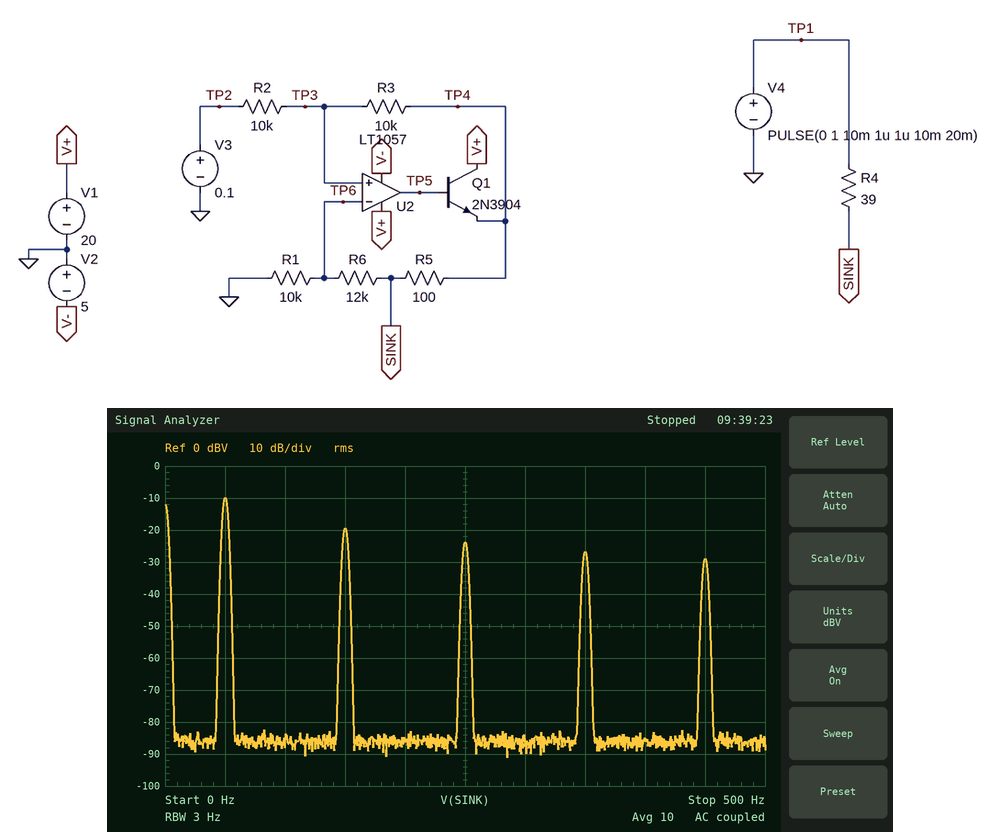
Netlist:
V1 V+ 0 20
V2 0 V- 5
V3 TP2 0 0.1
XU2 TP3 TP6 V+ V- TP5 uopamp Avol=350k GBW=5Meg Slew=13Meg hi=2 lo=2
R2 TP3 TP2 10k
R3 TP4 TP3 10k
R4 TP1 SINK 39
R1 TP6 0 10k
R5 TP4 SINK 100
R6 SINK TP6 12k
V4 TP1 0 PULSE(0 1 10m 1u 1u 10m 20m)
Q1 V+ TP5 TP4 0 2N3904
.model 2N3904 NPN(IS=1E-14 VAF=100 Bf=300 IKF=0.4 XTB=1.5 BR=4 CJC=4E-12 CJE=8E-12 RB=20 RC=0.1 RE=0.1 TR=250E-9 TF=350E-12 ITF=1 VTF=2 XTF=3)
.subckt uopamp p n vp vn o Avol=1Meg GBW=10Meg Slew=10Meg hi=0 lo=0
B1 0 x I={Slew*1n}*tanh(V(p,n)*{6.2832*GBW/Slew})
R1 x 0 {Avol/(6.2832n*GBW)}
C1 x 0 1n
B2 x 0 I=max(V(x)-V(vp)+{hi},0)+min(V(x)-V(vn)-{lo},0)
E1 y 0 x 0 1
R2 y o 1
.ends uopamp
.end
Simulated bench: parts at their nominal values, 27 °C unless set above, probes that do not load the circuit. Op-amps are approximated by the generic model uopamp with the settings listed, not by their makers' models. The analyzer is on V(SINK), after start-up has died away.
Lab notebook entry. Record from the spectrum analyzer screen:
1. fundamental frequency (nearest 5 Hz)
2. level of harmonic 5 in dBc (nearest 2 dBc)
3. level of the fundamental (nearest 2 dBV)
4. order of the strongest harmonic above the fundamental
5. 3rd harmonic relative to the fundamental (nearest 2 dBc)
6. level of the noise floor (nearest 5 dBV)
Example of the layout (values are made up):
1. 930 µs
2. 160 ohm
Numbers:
1. 50 Hz
2. -14 dBc
3. -10 dBV
4. 3
5. -10 dBc
6. -85 dBV
